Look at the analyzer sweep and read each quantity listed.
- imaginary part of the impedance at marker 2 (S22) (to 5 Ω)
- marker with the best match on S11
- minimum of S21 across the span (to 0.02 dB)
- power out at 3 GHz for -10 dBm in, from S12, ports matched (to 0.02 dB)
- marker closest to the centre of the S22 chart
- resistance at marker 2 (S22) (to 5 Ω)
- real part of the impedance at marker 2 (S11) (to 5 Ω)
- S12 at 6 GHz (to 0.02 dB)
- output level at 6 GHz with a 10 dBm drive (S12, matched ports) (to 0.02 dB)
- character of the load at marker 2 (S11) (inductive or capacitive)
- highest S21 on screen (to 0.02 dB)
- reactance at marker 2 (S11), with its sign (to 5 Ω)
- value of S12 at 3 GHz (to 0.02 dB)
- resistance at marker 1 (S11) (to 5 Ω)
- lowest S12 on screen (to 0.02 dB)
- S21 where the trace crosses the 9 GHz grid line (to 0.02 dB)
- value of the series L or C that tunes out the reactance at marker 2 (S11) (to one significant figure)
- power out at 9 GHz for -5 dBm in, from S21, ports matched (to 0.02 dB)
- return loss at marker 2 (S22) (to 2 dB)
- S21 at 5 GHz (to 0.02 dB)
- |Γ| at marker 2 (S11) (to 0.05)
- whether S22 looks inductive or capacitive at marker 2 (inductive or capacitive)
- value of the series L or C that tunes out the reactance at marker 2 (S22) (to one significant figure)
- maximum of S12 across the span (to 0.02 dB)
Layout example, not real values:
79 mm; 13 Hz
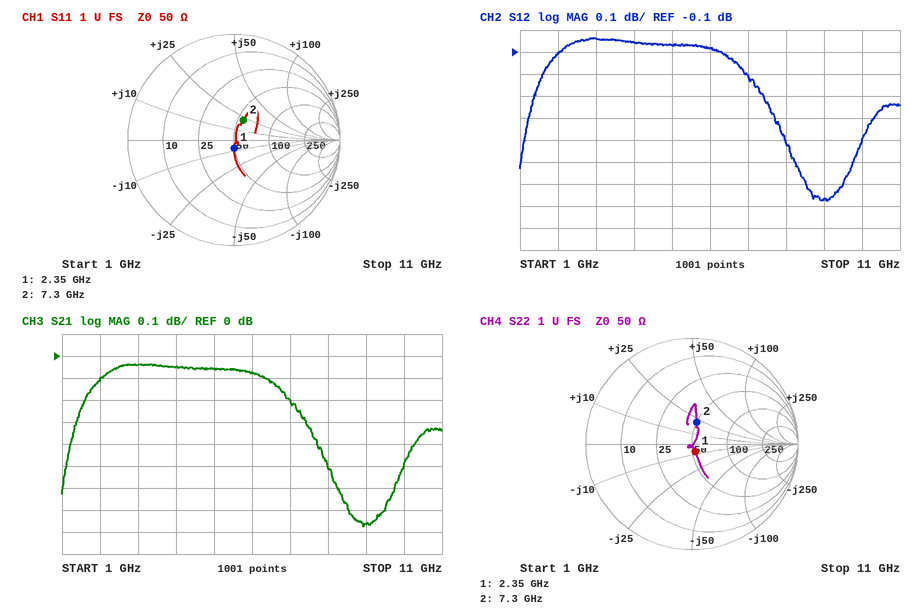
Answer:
+20 Ω; marker 1; -0.78 dB; -10.04 dBm; marker 1; 50 Ω; 55 Ω; -0.08 dB; 9.92 dBm; inductive; -0.04 dB; +20 Ω; -0.04 dB; 50 Ω; -0.78 dB; -0.76 dB; 1 pF; -5.76 dBm; 14 dB; -0.06 dB; 0.20; inductive; 1 pF; -0.04 dB
